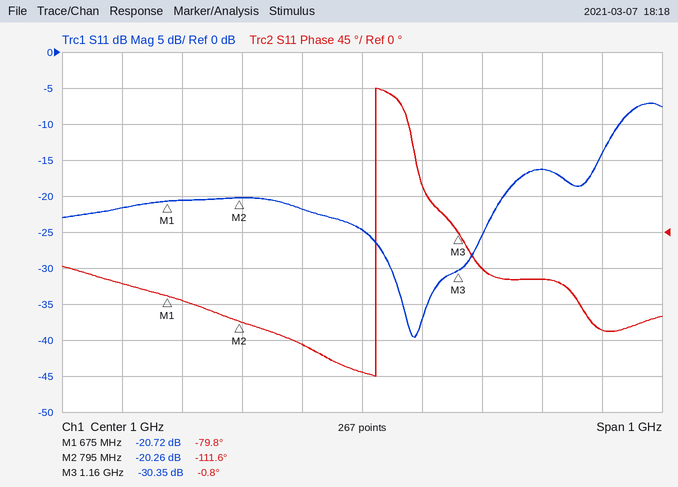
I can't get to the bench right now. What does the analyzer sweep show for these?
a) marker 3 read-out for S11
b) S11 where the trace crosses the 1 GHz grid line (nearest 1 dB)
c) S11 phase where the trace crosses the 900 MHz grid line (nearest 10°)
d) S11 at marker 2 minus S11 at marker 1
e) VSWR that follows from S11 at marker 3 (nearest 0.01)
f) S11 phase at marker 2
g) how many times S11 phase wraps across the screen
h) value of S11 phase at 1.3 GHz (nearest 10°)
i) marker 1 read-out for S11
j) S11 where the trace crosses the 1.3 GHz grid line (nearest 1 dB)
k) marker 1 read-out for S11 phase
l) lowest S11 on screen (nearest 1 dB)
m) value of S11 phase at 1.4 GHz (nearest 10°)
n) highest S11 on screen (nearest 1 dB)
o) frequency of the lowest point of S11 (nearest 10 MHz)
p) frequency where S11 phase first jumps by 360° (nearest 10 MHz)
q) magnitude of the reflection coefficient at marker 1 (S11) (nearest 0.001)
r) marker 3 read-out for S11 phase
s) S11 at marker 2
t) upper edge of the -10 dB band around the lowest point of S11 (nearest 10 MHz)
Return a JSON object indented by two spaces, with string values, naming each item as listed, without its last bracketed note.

{
  "marker 3 read-out for S11": "-30.35 dB",
  "S11 where the trace crosses the 1 GHz grid line": "-25 dB",
  "S11 phase where the trace crosses the 900 MHz grid line": "-140°",
  "S11 at marker 2 minus S11 at marker 1": "0.46 dB",
  "VSWR that follows from S11 at marker 3": "1.06",
  "S11 phase at marker 2": "-111.6°",
  "how many times S11 phase wraps across the screen": "1",
  "value of S11 phase at 1.3 GHz": "-60°",
  "marker 1 read-out for S11": "-20.72 dB",
  "S11 where the trace crosses the 1.3 GHz grid line": "-16 dB",
  "marker 1 read-out for S11 phase": "-79.8°",
  "lowest S11 on screen": "-40 dB",
  "value of S11 phase at 1.4 GHz": "-120°",
  "highest S11 on screen": "-7 dB",
  "frequency of the lowest point of S11": "1.09 GHz",
  "frequency where S11 phase first jumps by 360°": "1.02 GHz",
  "magnitude of the reflection coefficient at marker 1 (S11)": "0.092",
  "marker 3 read-out for S11 phase": "-0.8°",
  "S11 at marker 2": "-20.26 dB",
  "upper edge of the -10 dB band around the lowest point of S11": "1.43 GHz"
}
